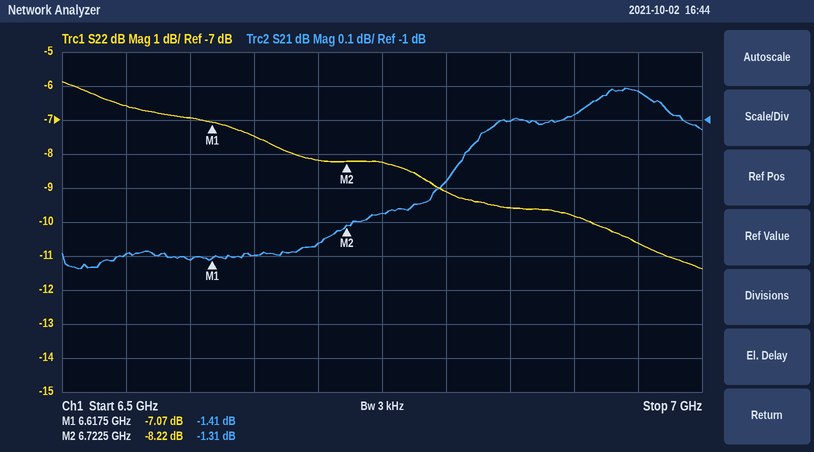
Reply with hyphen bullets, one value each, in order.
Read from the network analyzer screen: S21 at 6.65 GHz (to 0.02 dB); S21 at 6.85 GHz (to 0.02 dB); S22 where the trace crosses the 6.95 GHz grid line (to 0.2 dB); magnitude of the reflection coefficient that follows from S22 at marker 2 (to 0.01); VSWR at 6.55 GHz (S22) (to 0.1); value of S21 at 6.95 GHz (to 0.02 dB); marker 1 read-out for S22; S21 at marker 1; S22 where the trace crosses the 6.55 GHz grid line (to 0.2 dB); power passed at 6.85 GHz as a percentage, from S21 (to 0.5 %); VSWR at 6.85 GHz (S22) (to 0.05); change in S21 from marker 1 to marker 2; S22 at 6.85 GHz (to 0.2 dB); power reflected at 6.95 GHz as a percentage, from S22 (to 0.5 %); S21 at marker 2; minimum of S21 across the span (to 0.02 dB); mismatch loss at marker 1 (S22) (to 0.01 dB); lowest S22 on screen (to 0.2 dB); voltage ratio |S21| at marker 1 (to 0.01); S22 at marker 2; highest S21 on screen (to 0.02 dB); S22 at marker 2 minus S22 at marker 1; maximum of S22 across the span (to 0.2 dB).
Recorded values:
- -1.40 dB
- -1.00 dB
- -10.6 dB
- 0.39
- 2.8
- -0.92 dB
- -7.07 dB
- -1.41 dB
- -6.6 dB
- 79.5 %
- 2.00
- 0.10 dB
- -9.6 dB
- 8.5 %
- -1.31 dB
- -1.44 dB
- 0.95 dB
- -11.4 dB
- 0.85
- -8.22 dB
- -0.90 dB
- -1.15 dB
- -5.8 dB
